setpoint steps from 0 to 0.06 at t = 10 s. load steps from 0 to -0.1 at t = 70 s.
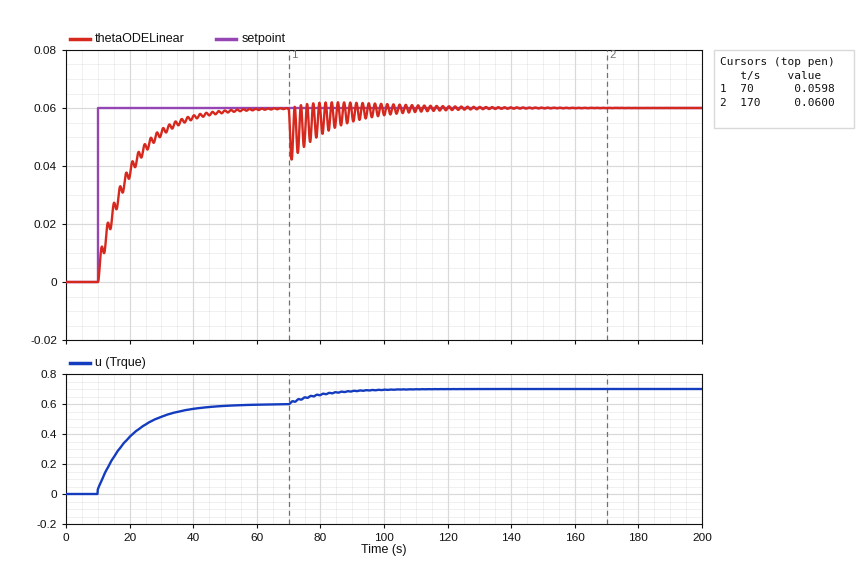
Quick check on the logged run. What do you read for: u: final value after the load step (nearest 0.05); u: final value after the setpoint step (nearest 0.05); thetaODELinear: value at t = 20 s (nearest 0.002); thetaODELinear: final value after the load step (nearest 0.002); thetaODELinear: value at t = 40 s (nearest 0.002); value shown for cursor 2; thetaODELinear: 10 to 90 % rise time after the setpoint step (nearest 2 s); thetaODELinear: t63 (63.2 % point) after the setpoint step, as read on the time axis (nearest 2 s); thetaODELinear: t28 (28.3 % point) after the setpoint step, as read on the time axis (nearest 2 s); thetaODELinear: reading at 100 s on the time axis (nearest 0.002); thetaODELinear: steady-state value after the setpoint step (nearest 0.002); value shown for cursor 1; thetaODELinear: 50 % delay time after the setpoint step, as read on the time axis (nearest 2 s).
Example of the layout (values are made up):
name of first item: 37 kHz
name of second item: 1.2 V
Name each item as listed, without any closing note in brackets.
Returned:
u: final value after the load step: 0.70
u: final value after the setpoint step: 0.60
thetaODELinear: value at t = 20 s: 0.036
thetaODELinear: final value after the load step: 0.060
thetaODELinear: value at t = 40 s: 0.058
value shown for cursor 2: 0.0600
thetaODELinear: 10 to 90 % rise time after the setpoint step: 22 s
thetaODELinear: t63 (63.2 % point) after the setpoint step, as read on the time axis: 20 s
thetaODELinear: t28 (28.3 % point) after the setpoint step, as read on the time axis: 12 s
thetaODELinear: reading at 100 s on the time axis: 0.058
thetaODELinear: steady-state value after the setpoint step: 0.060
value shown for cursor 1: 0.0598
thetaODELinear: 50 % delay time after the setpoint step, as read on the time axis: 16 s
